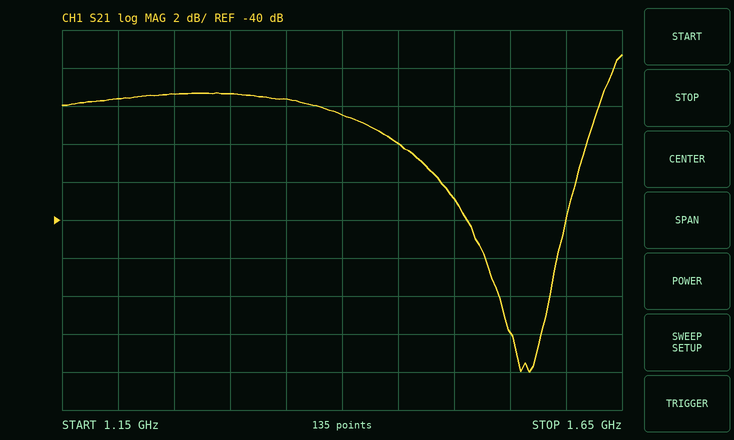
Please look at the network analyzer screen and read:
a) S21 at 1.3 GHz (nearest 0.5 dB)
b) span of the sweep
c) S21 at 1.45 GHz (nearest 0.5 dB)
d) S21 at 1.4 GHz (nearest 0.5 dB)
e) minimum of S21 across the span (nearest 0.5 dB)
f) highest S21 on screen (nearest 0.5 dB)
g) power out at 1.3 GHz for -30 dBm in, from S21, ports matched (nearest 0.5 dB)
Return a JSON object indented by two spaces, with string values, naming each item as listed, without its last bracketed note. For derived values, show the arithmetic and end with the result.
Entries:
{
  "S21 at 1.3 GHz": "-33.5 dB",
  "span of the sweep": "500 MHz",
  "S21 at 1.45 GHz": "-36.0 dB",
  "S21 at 1.4 GHz": "-34.5 dB",
  "minimum of S21 across the span": "-48.0 dB",
  "highest S21 on screen": "-31.5 dB",
  "power out at 1.3 GHz for -30 dBm in, from S21, ports matched": "-30 dBm + (-33.5 dB) = -63.5 dBm"
}
